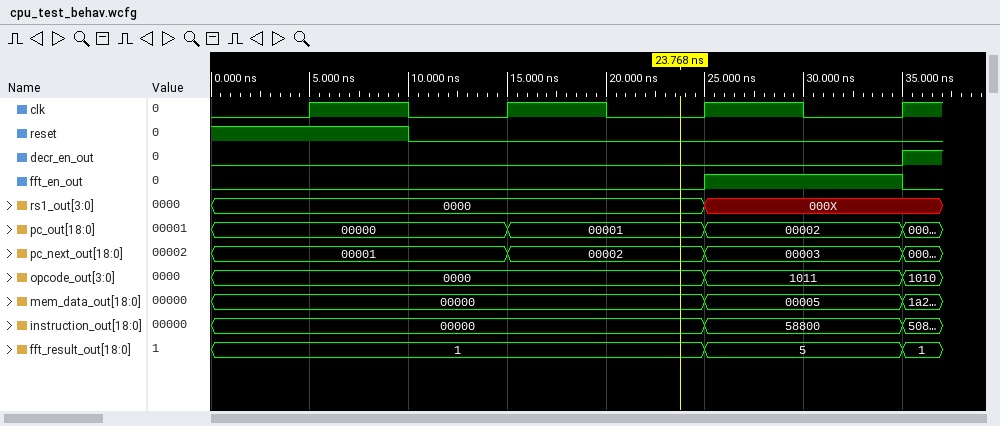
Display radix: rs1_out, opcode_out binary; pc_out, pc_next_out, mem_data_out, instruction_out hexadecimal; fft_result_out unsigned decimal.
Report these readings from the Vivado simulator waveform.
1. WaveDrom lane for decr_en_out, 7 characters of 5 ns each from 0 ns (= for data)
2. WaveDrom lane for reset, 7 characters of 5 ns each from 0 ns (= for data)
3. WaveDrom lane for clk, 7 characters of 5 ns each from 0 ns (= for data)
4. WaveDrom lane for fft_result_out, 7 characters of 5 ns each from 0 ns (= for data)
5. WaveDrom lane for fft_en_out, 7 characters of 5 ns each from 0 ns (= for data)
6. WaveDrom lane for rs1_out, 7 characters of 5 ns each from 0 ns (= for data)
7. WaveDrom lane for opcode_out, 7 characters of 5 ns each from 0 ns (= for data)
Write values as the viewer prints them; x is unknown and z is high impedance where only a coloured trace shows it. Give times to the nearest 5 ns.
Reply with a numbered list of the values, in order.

1. {name: 'decr_en_out', wave: '0......'}
2. {name: 'reset', wave: '1.0....'}
3. {name: 'clk', wave: '0101010'}
4. {name: 'fft_result_out', wave: '=....=.', data: '1 5'}
5. {name: 'fft_en_out', wave: '0....1.'}
6. {name: 'rs1_out', wave: '=....=.', data: '0000 000X'}
7. {name: 'opcode_out', wave: '=....=.', data: '0000 1011'}
